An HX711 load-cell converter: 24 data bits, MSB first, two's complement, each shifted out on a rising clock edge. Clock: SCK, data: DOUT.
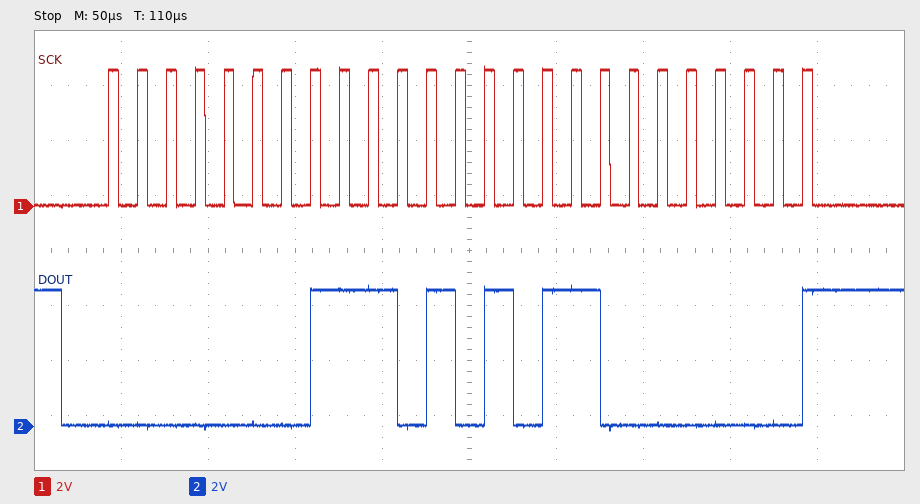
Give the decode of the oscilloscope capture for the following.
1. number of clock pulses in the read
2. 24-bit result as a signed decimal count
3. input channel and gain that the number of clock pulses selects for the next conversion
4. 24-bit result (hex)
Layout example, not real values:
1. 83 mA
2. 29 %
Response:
1. 25
2. 120192
3. channel A, gain 128
4. 0x01D580
